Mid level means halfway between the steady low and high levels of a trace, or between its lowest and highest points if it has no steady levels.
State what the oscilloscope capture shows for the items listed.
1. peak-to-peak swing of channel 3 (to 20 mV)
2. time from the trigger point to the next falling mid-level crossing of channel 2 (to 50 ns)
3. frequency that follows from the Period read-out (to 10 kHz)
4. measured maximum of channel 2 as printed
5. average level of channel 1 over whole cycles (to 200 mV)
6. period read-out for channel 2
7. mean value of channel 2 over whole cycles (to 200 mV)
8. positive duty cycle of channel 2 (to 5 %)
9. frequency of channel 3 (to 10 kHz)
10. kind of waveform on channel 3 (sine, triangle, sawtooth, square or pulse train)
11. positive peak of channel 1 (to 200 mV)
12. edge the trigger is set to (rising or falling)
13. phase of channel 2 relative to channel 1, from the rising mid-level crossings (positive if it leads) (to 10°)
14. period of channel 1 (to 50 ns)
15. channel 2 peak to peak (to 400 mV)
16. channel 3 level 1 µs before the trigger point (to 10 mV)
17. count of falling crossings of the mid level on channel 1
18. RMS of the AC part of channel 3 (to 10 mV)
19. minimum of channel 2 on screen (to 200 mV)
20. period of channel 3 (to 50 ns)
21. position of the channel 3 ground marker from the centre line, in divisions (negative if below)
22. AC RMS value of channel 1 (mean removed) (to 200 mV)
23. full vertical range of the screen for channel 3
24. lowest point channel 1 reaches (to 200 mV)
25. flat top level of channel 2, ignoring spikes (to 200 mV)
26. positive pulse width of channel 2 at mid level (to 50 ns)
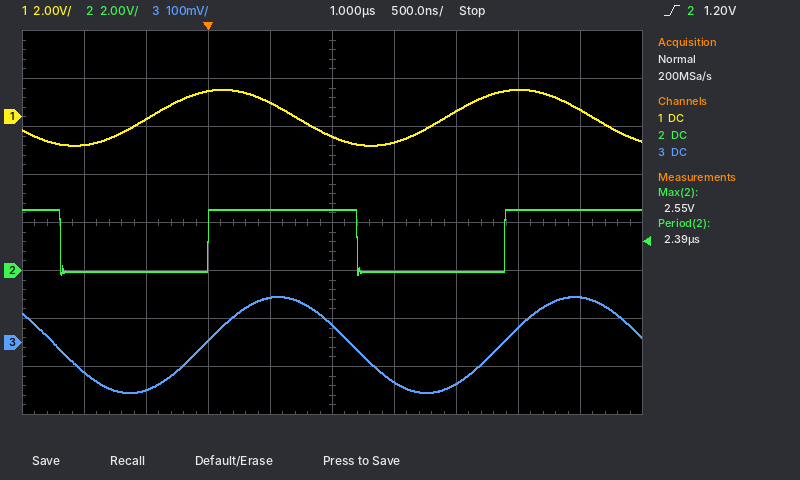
200 mV
1.20 µs
420 kHz
2.55 V
0.0 V
2.39 µs
1.2 V
50 %
420 kHz
sine
1.2 V
rising
-70°
2.40 µs
2.8 V
-60 mV
2
70 mV
-200 mV
2.40 µs
-2.5 div
800 mV
800 mV
-1.2 V
2.6 V
1.20 µs
